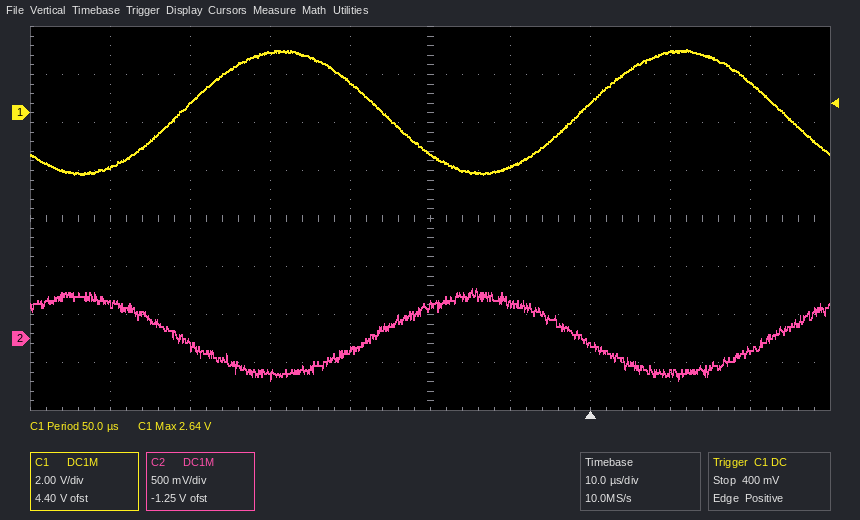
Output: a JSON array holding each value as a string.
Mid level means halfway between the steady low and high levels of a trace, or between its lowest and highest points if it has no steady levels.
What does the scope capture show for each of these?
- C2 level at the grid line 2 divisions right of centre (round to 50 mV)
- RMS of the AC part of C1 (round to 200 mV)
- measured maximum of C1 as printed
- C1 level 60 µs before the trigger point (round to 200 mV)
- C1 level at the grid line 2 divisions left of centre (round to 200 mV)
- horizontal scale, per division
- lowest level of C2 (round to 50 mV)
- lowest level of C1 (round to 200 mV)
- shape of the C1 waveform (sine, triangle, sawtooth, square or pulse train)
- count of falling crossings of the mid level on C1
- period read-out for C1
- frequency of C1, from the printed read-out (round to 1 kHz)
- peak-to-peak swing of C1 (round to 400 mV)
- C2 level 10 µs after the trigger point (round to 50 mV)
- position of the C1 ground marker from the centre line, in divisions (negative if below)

["-50 mV", "1.8 V", "2.64 V", "-2.2 V", "2.6 V", "10 µs", "-450 mV", "-2.6 V", "sine", "2", "50.0 µs", "20 kHz", "5.2 V", "-350 mV", "+2.2 div"]
